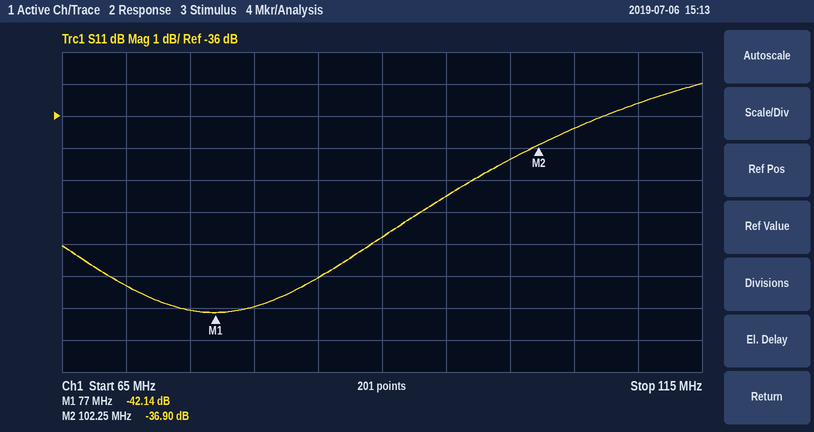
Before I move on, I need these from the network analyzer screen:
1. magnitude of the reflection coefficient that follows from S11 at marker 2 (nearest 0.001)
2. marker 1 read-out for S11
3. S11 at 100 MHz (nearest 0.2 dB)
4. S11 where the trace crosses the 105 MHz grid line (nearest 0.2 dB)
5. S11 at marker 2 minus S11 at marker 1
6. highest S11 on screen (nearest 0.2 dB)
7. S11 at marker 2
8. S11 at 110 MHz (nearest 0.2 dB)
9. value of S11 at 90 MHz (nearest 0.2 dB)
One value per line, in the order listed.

0.014
-42.14 dB
-37.4 dB
-36.4 dB
5.24 dB
-35.0 dB
-36.90 dB
-35.6 dB
-39.8 dB
